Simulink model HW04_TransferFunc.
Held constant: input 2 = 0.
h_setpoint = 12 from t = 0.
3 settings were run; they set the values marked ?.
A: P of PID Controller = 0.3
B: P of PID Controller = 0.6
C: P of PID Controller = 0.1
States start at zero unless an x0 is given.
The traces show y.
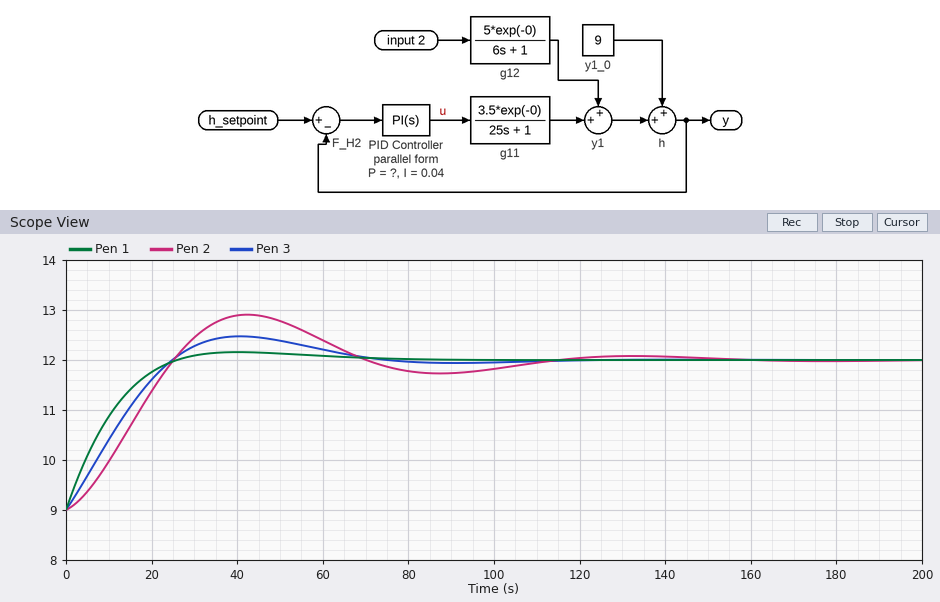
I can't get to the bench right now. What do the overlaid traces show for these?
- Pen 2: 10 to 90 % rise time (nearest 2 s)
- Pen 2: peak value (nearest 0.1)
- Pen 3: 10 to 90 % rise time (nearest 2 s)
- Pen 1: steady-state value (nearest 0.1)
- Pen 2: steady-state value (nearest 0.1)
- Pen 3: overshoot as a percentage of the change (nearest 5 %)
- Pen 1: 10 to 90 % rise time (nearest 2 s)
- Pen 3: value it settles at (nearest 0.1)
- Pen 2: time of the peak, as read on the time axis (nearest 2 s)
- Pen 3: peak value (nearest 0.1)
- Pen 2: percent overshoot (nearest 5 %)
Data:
18 s
12.9
18 s
12.0
12.0
15 %
18 s
12.0
42 s
12.5
30 %
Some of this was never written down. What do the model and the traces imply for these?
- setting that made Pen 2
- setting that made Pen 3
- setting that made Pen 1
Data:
C
A
B
